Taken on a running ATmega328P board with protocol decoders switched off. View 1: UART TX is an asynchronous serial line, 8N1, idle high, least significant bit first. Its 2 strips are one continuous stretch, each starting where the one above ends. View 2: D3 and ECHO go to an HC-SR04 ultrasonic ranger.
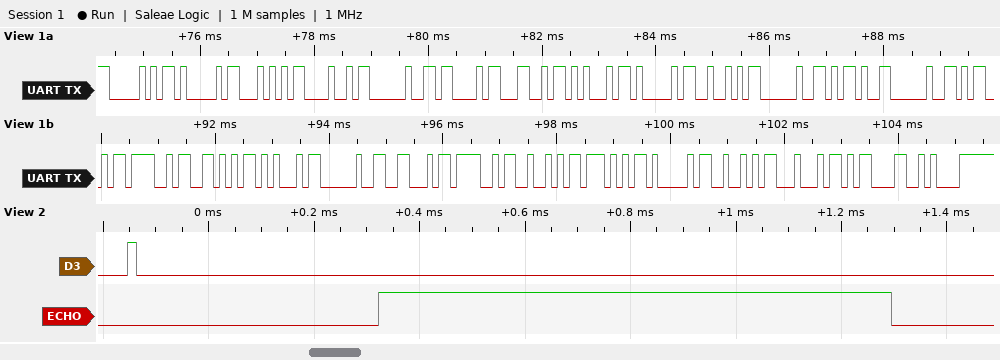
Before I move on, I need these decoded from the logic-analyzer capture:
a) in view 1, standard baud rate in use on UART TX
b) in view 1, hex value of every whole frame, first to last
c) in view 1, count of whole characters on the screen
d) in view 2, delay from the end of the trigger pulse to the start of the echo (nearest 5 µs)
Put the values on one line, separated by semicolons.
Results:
9600 baud; 0x50 0x41 0x54 0x48 0x20 0x43 0x4C 0x45 0x41 0x52 0x20 0x2D 0x20 0x4D 0x4F 0x56 0x45 0x20 0x46 0x4F 0x52 0x57 0x41 0x52 0x44 0x0D 0x0A; 27; 460 µs
